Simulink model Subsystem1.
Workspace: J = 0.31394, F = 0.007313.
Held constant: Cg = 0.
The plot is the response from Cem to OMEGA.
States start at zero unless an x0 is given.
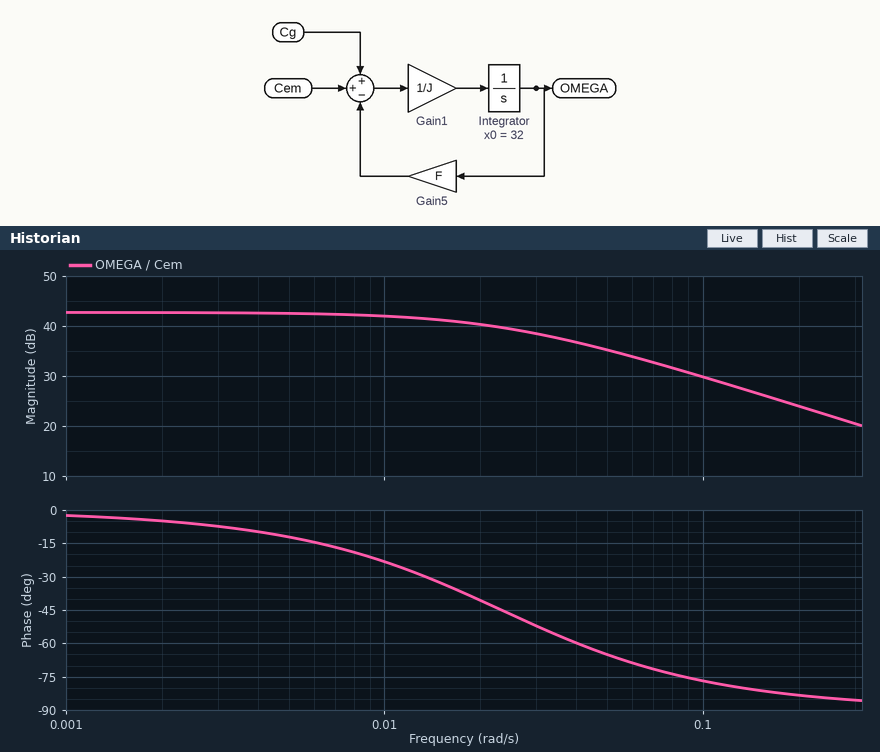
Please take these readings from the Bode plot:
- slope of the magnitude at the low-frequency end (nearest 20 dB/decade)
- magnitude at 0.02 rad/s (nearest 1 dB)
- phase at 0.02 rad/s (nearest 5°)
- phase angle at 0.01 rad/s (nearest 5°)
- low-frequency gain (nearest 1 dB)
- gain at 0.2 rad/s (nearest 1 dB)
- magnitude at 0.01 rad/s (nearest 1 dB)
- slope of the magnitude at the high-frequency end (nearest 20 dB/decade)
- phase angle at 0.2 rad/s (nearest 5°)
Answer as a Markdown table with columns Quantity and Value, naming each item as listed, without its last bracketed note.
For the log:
| Quantity | Value |
|---|---|
| slope of the magnitude at the low-frequency end | 0 dB/decade |
| magnitude at 0.02 rad/s | 40 dB |
| phase at 0.02 rad/s | -40° |
| phase angle at 0.01 rad/s | -25° |
| low-frequency gain | 43 dB |
| gain at 0.2 rad/s | 24 dB |
| magnitude at 0.01 rad/s | 42 dB |
| slope of the magnitude at the high-frequency end | -20 dB/decade |
| phase angle at 0.2 rad/s | -85° |
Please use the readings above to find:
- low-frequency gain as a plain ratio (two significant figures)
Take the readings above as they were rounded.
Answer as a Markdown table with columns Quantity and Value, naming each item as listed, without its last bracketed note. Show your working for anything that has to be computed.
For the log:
| Quantity | Value |
|---|---|
| low-frequency gain as a plain ratio | 10^(43 / 20) = 140 |
